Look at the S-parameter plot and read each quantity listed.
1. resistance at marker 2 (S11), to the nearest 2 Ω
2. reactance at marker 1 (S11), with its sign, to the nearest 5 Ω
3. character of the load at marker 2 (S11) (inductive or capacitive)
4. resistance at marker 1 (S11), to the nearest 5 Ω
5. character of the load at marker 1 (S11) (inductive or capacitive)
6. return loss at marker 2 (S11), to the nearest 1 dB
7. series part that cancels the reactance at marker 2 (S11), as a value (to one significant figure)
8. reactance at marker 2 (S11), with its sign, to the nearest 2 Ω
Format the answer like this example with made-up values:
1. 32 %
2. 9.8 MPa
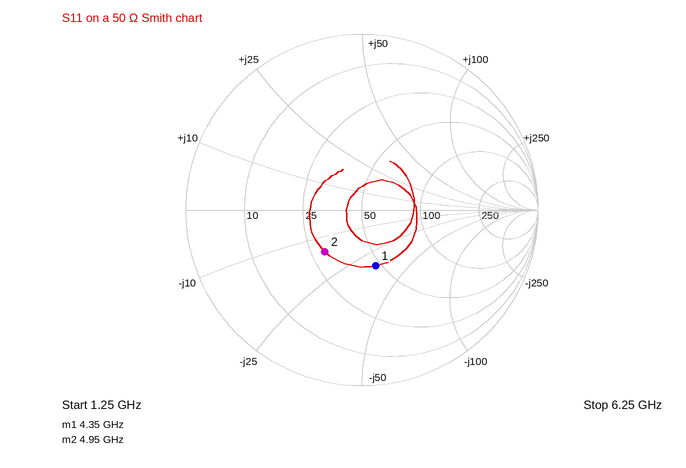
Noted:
1. 30 Ω
2. -35 Ω
3. capacitive
4. 45 Ω
5. capacitive
6. 10 dB
7. 500 pH
8. -16 Ω
